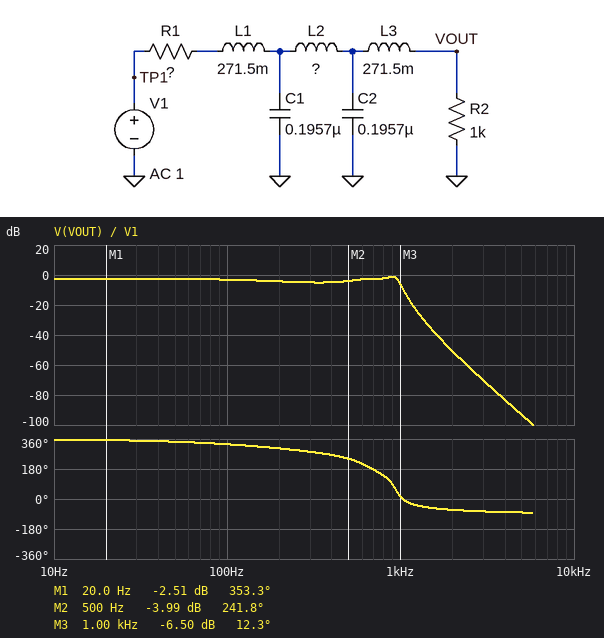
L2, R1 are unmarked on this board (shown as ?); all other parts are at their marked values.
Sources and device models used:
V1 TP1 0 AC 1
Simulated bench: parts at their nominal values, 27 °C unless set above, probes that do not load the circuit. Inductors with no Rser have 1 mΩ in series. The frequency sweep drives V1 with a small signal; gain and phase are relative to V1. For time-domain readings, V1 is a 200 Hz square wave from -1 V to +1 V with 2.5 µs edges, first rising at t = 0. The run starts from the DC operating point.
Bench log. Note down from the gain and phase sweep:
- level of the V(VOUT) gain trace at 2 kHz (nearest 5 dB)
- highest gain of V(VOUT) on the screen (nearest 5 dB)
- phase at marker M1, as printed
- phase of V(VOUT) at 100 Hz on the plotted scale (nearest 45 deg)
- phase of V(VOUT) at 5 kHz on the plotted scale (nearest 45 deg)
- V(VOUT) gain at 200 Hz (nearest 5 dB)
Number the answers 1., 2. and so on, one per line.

1. -50 dB
2. 0 dB
3. 353.3 deg
4. 315 deg
5. -90 deg
6. -5 dB
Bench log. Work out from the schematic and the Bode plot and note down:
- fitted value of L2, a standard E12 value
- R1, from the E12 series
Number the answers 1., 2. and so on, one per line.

1. 560 mH
2. 330 Ω
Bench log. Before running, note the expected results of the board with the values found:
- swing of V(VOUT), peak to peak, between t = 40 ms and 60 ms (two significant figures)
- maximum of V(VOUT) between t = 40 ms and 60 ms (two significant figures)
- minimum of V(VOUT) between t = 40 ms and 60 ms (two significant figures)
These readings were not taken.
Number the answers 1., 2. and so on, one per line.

1. 1.6 V
2. 810 mV
3. -810 mV
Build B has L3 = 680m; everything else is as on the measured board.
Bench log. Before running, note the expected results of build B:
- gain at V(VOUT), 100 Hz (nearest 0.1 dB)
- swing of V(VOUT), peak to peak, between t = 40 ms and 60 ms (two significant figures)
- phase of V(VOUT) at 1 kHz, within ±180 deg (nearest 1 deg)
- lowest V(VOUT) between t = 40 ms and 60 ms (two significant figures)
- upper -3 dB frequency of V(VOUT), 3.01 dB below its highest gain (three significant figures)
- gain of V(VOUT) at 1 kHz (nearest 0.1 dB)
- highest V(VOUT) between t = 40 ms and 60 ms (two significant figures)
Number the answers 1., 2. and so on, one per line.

1. -3.8 dB
2. 1.5 V
3. -38 deg
4. -740 mV
5. 620 Hz
6. -15.1 dB
7. 740 mV
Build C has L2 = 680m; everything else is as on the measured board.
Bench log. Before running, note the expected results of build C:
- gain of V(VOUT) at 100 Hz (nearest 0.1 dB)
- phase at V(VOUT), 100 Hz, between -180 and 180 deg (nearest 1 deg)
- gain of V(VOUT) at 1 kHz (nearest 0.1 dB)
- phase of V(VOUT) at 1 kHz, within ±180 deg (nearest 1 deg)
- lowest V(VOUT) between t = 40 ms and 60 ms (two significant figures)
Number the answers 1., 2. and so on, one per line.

1. -3.3 dB
2. -34 deg
3. -10.7 dB
4. -1 deg
5. -790 mV
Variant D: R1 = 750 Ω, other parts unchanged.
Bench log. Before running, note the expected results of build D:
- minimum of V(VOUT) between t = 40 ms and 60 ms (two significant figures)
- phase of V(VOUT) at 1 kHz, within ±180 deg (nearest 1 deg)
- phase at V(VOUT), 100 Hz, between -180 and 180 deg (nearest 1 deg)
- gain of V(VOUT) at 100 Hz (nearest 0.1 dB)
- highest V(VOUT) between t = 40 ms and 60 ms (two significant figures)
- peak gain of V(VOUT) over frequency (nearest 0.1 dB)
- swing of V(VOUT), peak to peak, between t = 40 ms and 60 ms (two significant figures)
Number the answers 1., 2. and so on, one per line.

1. -670 mV
2. 31 deg
3. -28 deg
4. -5.2 dB
5. 670 mV
6. -4.8 dB
7. 1.3 V
